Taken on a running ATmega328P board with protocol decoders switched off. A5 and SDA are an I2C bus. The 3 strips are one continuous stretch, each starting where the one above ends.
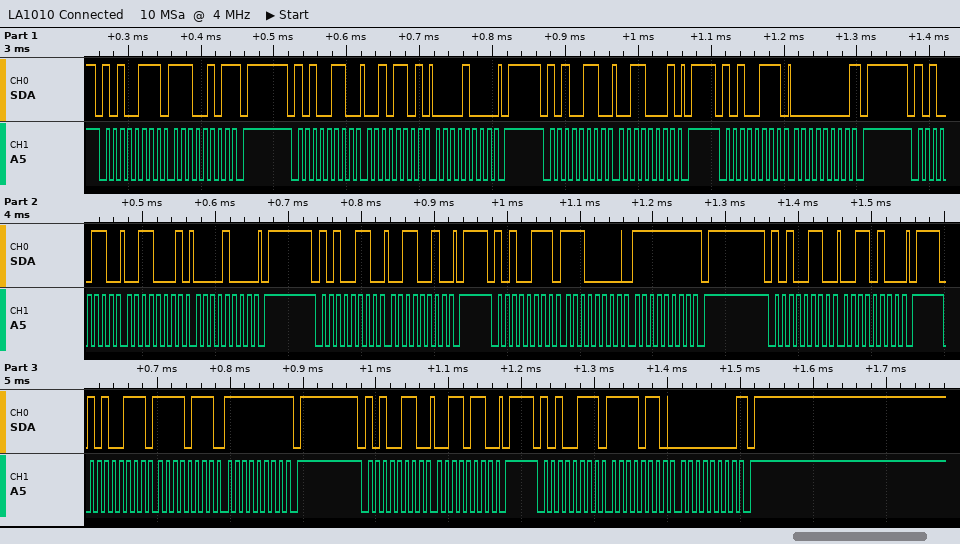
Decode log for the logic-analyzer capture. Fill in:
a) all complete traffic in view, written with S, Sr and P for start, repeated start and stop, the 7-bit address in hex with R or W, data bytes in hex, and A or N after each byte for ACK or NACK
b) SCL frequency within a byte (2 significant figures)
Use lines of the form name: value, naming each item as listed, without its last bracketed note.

all complete traffic in view, written with S, Sr and P for start, repeated start and stop, the 7-bit address in hex with R or W, data bytes in hex, and A or N after each byte for ACK or NACK: S 53R A E5 N P S 53W A 2D A 08 A P S 53W A 31 A P S 53R A 00 N P S 53W A 31 A 08 A P S 53W A 32 A P S 53R A E0 A FF N P S 53W A 34 A P S 53R A F7 A FF N P S 53W A 36 A P S 53R A F6 A 00 N P
SCL frequency within a byte: 100 kHz
